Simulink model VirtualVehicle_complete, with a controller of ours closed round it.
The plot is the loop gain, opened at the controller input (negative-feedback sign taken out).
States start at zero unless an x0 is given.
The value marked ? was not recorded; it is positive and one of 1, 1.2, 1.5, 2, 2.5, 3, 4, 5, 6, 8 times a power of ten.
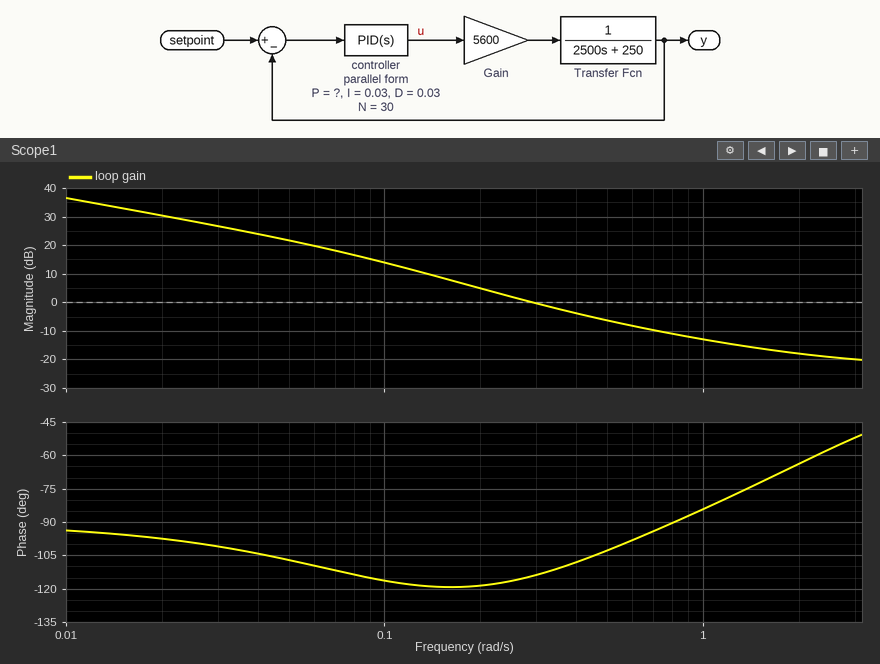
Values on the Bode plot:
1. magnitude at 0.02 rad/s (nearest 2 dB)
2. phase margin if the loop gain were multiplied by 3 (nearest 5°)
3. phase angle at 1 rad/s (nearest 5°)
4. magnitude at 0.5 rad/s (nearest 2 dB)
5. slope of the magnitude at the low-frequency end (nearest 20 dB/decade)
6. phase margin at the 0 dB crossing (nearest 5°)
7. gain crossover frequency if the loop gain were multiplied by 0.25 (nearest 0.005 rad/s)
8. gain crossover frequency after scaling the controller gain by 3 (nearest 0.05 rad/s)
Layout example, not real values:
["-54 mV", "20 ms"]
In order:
["30 dB", "85°", "-85°", "-6 dB", "-20 dB/decade", "65°", "0.115 rad/s", "0.70 rad/s"]
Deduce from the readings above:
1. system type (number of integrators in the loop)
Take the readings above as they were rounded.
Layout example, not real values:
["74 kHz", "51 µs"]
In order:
["1"]
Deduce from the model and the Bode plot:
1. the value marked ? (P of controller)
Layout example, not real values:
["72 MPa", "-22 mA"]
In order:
["0.1"]
